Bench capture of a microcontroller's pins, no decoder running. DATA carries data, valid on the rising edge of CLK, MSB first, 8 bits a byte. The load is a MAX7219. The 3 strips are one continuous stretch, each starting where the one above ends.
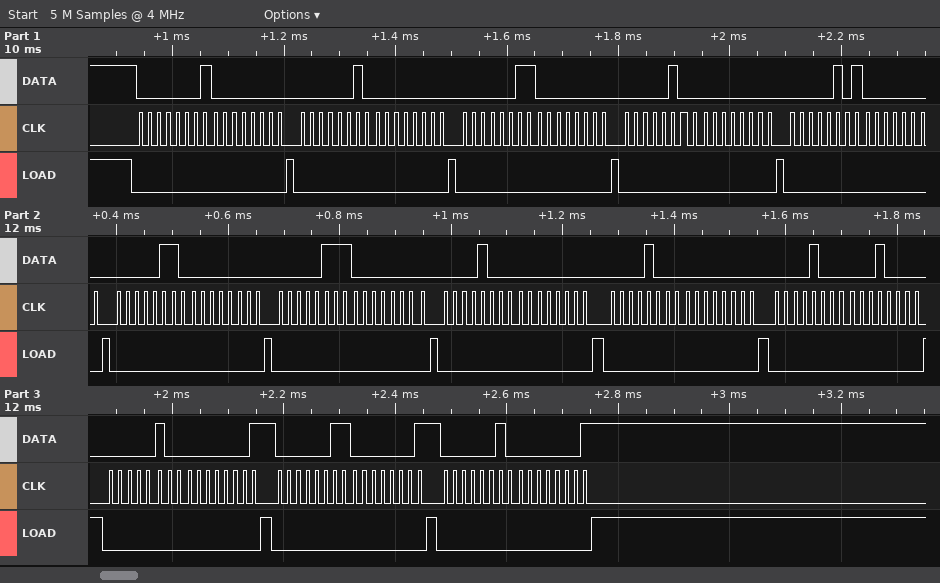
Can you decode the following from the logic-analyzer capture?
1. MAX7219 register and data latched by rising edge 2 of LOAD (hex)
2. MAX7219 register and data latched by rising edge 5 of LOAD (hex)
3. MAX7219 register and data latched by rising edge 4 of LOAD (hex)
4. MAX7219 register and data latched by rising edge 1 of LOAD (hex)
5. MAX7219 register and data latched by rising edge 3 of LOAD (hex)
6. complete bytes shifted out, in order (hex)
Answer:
register 0x2, data 0x00
register 0x5, data 0x00
register 0x4, data 0x00
register 0x1, data 0x00
register 0x3, data 0x00
01 00 02 00 03 00 04 00 05 00 06 00 07 00 08 00 08 00 08 10 04 01 03 01 02 01
